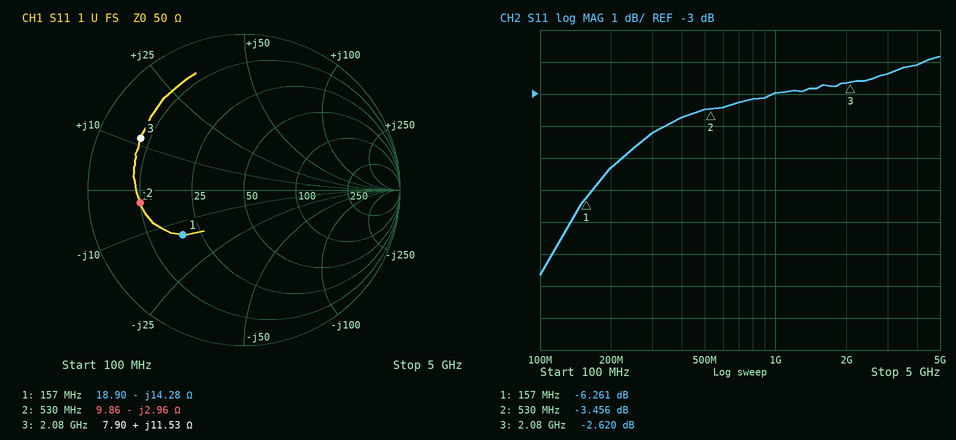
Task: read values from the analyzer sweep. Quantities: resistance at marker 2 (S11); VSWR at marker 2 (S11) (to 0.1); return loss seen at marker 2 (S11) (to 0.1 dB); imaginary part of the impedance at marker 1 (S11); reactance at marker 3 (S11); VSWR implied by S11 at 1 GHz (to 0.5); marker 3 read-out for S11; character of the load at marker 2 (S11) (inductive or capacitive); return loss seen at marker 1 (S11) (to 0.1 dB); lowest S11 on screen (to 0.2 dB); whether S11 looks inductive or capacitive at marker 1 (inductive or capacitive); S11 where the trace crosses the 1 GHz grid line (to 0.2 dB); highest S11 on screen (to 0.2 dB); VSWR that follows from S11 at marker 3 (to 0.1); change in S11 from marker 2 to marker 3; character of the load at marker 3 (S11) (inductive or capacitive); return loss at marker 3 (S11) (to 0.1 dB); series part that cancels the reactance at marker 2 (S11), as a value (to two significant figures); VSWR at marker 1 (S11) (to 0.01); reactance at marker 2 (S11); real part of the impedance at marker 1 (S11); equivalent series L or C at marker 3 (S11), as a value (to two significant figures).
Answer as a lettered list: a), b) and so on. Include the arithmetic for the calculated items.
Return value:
a) 9.86 Ω
b) (1 + 0.6717)/(1 − 0.6717) ≈ 5.1
c) 3.5 dB
d) -14.28 Ω
e) +11.53 Ω
f) |Γ| = 10^(-3/20) = 0.7079; VSWR = (1 + 0.7079)/(1 − 0.7079) ≈ 5.85, so 6.0 to the nearest 0.5
g) -2.620 dB
h) capacitive
i) 6.3 dB
j) -8.6 dB
k) capacitive
l) -3.0 dB
m) -1.8 dB
n) (1 + 0.7396)/(1 − 0.7396) ≈ 6.7
o) -2.62 − (-3.456) = 0.836 dB
p) inductive
q) 2.6 dB
r) L = 2.96 Ω/(2π × 530 MHz) ≈ 889 pH, so 890 pH to two significant figures
s) (1 + 0.4864)/(1 − 0.4864) ≈ 2.89
t) -2.96 Ω
u) 18.90 Ω
v) L = 11.53 Ω/(2π × 2.08 GHz) ≈ 882 pH, so 880 pH to two significant figures
